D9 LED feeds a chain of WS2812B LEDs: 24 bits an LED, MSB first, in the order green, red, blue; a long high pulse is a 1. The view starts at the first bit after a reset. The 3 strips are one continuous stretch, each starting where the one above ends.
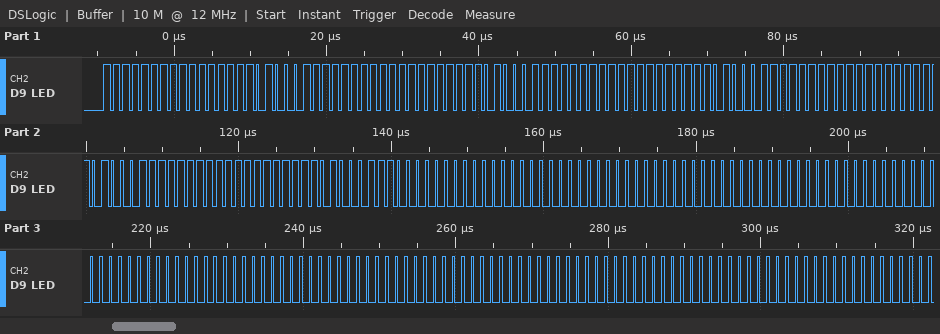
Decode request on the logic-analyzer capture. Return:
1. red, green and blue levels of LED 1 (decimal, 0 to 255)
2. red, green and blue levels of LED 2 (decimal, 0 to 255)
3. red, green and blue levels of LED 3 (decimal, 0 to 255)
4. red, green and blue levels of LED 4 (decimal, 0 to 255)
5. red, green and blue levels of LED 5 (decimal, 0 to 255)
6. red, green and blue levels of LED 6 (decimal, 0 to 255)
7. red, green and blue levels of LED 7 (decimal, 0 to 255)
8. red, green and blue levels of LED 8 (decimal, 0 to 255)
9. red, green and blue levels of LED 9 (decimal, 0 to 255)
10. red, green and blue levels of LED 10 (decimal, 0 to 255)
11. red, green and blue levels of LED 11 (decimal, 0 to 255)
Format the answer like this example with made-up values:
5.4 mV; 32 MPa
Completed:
255, 255, 71; 255, 255, 71; 255, 255, 71; 255, 255, 71; 255, 255, 71; 0, 0, 0; 0, 0, 0; 0, 0, 0; 0, 0, 0; 0, 0, 0; 0, 0, 0
